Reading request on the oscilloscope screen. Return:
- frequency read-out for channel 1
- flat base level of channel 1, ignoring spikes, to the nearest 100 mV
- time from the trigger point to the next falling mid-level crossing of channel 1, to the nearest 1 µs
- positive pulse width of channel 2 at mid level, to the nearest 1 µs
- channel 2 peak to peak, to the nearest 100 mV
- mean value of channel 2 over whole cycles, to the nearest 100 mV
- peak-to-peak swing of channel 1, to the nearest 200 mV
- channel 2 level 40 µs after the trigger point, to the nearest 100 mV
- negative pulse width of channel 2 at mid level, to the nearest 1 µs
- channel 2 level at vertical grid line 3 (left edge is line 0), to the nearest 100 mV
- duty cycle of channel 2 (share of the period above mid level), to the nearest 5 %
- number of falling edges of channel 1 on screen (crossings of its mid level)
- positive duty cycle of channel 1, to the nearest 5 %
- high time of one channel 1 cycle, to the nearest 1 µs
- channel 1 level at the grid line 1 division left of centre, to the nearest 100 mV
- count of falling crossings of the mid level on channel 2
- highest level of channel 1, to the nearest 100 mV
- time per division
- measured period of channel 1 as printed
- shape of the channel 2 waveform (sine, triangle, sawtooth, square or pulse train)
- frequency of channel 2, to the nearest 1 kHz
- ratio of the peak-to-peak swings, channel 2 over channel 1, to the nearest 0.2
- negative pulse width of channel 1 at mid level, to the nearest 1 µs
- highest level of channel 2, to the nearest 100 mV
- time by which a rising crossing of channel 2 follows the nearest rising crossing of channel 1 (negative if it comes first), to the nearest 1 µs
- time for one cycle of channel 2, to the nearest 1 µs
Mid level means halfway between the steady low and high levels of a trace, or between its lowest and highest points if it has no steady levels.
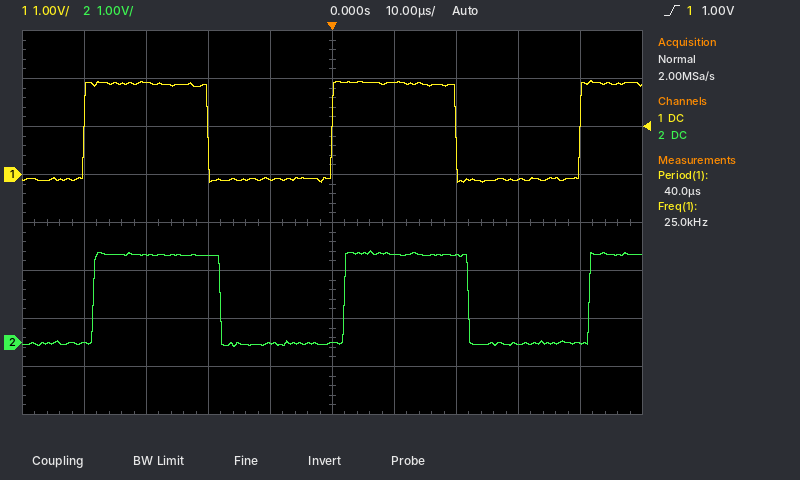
25.0 kHz
-100 mV
20 µs
20 µs
2.0 V
900 mV
2.2 V
0.0 V
20 µs
1.8 V
50 %
2
50 %
20 µs
-100 mV
2
2.0 V
10 µs
40.0 µs
square
25 kHz
1.0
20 µs
1.9 V
+2 µs
40 µs
